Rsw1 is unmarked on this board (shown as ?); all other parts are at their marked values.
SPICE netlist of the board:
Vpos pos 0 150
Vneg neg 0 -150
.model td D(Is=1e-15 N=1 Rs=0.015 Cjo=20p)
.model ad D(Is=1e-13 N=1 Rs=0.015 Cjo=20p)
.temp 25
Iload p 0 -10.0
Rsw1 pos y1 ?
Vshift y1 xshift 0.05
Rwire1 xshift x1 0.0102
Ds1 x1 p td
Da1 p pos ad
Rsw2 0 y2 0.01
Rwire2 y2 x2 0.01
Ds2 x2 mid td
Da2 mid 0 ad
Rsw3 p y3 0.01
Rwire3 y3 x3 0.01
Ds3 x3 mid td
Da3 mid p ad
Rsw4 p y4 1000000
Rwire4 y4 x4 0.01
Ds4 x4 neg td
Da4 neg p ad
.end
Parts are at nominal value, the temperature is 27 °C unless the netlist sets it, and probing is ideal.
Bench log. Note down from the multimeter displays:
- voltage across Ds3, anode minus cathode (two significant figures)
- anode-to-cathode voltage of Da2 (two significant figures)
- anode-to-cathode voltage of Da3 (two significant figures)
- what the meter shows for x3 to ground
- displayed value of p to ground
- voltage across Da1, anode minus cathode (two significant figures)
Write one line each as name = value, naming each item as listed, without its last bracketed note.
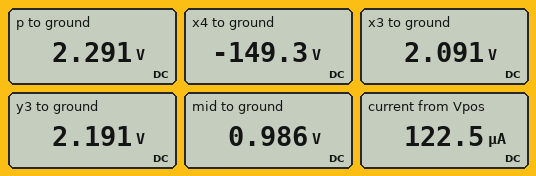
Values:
voltage across Ds3, anode minus cathode = 1.1 V
anode-to-cathode voltage of Da2 = 990 mV
anode-to-cathode voltage of Da3 = -1.3 V
what the meter shows for x3 to ground = 2.091 V
displayed value of p to ground = 2.291 V
voltage across Da1, anode minus cathode = -150 V
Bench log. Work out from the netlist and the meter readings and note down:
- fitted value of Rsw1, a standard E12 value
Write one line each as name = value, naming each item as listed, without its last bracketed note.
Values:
fitted value of Rsw1, a standard E12 value = 1.2 MΩ
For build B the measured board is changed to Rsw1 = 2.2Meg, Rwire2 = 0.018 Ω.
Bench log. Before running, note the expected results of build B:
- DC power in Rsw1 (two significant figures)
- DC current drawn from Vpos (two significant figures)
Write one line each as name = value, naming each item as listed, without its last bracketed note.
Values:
DC power in Rsw1 = 9.8 mW
DC current drawn from Vpos = 67 µA
